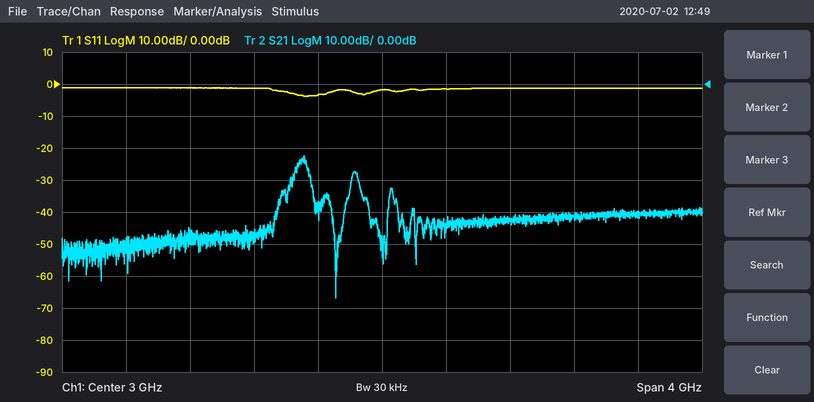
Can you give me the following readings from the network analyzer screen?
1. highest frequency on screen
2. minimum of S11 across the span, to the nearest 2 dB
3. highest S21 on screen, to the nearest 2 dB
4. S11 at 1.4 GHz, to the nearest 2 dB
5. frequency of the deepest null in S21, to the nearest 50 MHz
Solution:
5 GHz
-4 dB
-22 dB
-2 dB
2.70 GHz
